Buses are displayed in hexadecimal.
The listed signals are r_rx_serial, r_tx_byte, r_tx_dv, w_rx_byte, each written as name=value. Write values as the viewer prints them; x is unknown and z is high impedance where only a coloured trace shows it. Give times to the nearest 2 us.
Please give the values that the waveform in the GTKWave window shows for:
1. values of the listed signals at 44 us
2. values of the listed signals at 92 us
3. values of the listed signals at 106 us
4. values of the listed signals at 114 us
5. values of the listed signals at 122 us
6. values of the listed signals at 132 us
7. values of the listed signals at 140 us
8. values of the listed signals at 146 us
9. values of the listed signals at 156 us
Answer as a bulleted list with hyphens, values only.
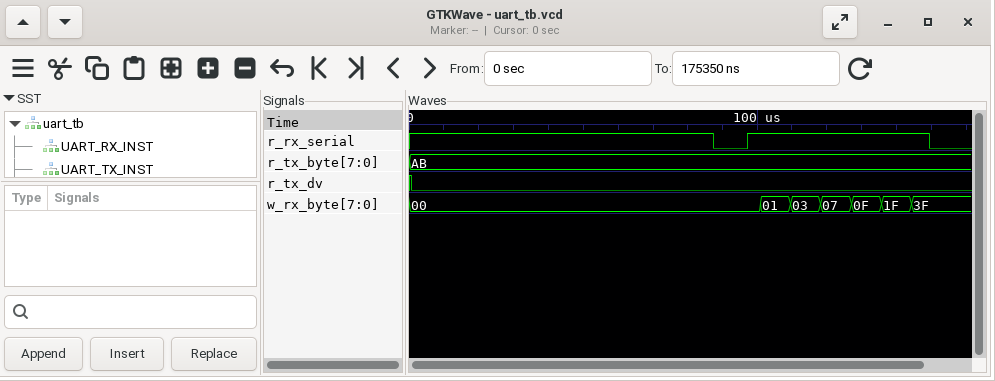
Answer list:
- r_rx_serial=1, r_tx_byte=AB, r_tx_dv=0, w_rx_byte=00
- r_rx_serial=0, r_tx_byte=AB, r_tx_dv=0, w_rx_byte=00
- r_rx_serial=1, r_tx_byte=AB, r_tx_dv=0, w_rx_byte=01
- r_rx_serial=1, r_tx_byte=AB, r_tx_dv=0, w_rx_byte=03
- r_rx_serial=1, r_tx_byte=AB, r_tx_dv=0, w_rx_byte=07
- r_rx_serial=1, r_tx_byte=AB, r_tx_dv=0, w_rx_byte=0F
- r_rx_serial=1, r_tx_byte=AB, r_tx_dv=0, w_rx_byte=1F
- r_rx_serial=1, r_tx_byte=AB, r_tx_dv=0, w_rx_byte=3F
- r_rx_serial=0, r_tx_byte=AB, r_tx_dv=0, w_rx_byte=3F
